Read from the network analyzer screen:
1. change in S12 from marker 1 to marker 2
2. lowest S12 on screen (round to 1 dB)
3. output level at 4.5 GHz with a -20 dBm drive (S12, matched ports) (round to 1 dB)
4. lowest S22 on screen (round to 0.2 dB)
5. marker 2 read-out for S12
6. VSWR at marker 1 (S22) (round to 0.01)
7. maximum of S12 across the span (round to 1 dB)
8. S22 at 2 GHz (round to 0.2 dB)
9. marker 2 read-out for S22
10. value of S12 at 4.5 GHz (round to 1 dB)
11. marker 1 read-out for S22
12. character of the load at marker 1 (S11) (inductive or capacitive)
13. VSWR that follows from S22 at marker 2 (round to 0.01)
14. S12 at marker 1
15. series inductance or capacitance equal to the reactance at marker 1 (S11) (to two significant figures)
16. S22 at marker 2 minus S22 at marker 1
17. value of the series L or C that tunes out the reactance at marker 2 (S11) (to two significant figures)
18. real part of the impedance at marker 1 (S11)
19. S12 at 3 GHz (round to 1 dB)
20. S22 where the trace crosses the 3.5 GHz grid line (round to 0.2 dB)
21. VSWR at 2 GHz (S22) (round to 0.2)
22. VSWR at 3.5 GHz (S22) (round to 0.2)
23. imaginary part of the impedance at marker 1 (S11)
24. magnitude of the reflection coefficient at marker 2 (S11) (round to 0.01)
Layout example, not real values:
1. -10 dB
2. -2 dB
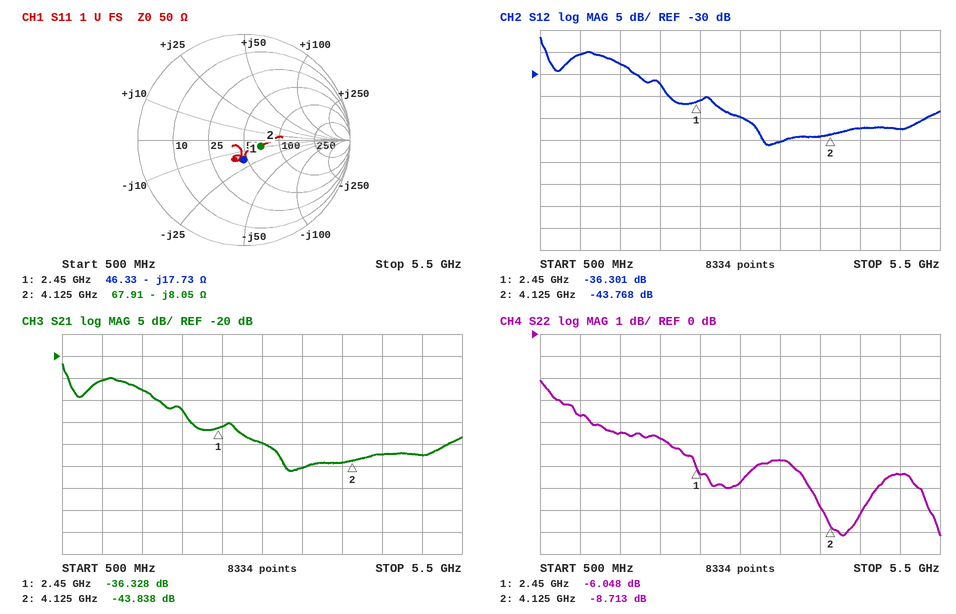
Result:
1. -7.467 dB
2. -46 dB
3. -62 dBm
4. -9.2 dB
5. -43.768 dB
6. 2.99
7. -22 dB
8. -4.8 dB
9. -8.713 dB
10. -42 dB
11. -6.048 dB
12. capacitive
13. 2.16
14. -36.301 dB
15. 3.7 pF
16. -2.665 dB
17. 310 pH
18. 46.33 Ω
19. -40 dB
20. -5.8 dB
21. 3.8
22. 3.2
23. -17.73 Ω
24. 0.17
